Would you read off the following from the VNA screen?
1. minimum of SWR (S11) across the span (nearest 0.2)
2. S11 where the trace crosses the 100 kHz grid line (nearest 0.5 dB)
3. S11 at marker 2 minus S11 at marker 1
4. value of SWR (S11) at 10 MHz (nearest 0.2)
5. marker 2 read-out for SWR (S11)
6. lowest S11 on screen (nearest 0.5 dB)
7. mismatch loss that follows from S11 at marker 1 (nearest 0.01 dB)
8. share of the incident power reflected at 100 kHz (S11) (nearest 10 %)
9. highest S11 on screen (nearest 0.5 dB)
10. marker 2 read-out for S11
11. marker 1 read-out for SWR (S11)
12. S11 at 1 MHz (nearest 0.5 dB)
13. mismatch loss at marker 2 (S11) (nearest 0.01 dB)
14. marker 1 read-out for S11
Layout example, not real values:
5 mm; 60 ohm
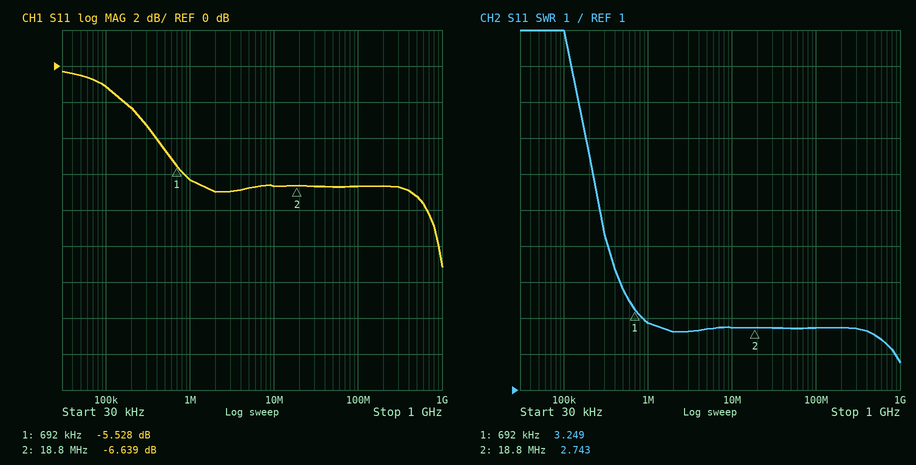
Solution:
1.8; -1.0 dB; -1.111 dB; 2.8; 2.743; -11.0 dB; 1.43 dB; 80 %; -0.5 dB; -6.639 dB; 3.249; -6.5 dB; 1.06 dB; -5.528 dB
